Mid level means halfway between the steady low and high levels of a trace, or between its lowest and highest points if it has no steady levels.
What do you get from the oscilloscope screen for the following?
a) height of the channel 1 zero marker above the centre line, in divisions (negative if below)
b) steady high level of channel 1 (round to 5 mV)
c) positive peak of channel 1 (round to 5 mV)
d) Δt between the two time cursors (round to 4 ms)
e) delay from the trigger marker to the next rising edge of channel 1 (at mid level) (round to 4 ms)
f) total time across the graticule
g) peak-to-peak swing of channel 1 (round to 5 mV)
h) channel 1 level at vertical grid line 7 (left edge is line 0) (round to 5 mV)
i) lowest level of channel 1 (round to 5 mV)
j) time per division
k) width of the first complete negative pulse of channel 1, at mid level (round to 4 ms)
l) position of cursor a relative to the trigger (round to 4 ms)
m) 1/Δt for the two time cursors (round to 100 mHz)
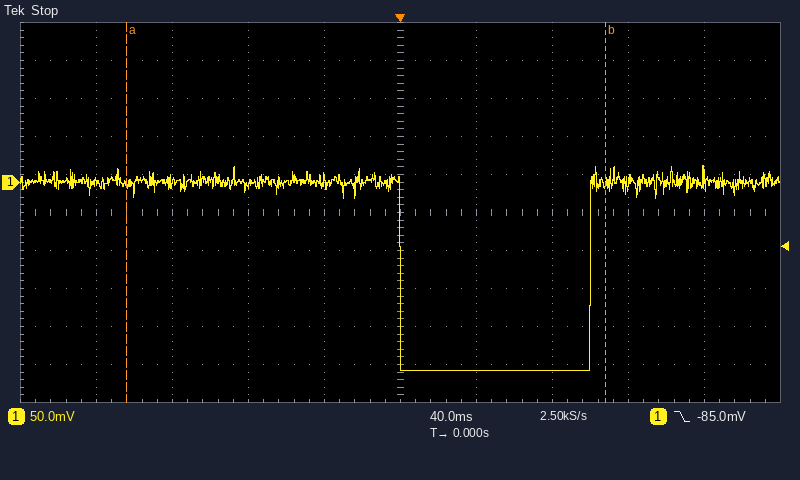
+0.8 div
0 mV
20 mV
252 ms
100 ms
400 ms
270 mV
-250 mV
-250 mV
40 ms
100 ms
-144 ms
4.0 Hz
